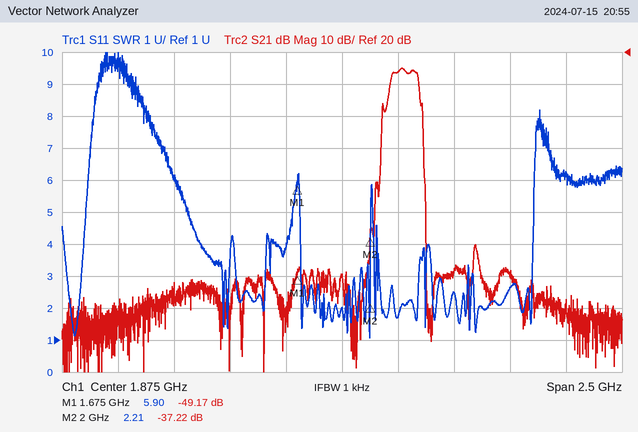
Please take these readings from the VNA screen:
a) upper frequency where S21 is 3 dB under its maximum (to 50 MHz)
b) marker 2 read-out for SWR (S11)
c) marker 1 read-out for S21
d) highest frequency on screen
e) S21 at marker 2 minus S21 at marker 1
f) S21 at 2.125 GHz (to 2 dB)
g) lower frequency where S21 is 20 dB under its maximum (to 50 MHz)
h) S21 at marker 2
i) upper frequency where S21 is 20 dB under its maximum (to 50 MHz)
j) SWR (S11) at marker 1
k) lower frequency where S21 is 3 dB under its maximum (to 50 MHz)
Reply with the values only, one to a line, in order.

2.20 GHz
2.21
-49.17 dB
3.125 GHz
11.95 dB
14 dB
2.05 GHz
-37.22 dB
2.25 GHz
5.90
2.10 GHz
